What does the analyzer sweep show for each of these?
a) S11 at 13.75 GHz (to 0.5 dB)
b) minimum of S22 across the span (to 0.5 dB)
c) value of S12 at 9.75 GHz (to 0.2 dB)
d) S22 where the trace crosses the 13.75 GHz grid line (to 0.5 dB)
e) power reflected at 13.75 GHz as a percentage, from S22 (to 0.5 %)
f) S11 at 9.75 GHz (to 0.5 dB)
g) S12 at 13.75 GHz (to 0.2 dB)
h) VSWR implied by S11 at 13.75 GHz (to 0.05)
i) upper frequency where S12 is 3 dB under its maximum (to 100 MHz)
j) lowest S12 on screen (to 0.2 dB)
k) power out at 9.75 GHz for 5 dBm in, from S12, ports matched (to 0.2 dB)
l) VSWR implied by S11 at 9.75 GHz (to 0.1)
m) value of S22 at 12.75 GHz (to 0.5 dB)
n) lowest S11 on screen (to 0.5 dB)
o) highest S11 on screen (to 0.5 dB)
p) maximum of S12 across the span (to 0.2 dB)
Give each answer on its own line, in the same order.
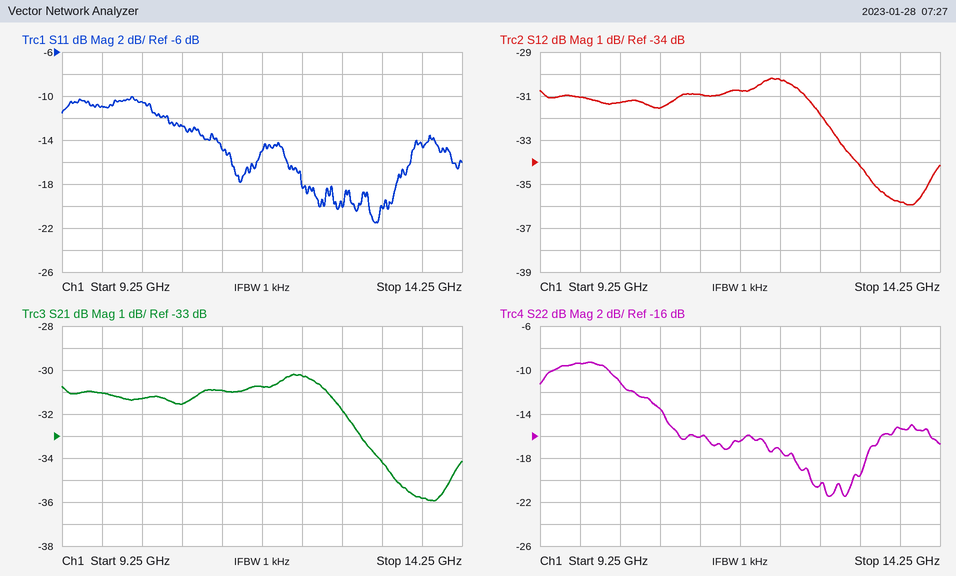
-14.5 dB
-21.5 dB
-31.0 dB
-15.5 dB
3.0 %
-11.0 dB
-35.8 dB
1.45
13.0 GHz
-36.0 dB
-26.0 dBm
1.8
-20.5 dB
-21.5 dB
-10.0 dB
-30.2 dB
